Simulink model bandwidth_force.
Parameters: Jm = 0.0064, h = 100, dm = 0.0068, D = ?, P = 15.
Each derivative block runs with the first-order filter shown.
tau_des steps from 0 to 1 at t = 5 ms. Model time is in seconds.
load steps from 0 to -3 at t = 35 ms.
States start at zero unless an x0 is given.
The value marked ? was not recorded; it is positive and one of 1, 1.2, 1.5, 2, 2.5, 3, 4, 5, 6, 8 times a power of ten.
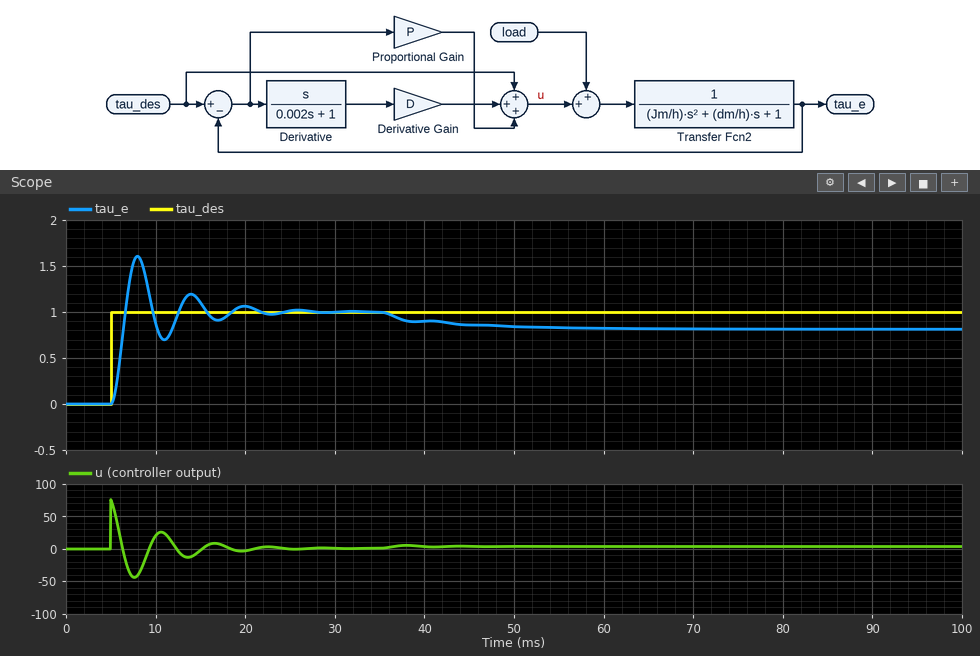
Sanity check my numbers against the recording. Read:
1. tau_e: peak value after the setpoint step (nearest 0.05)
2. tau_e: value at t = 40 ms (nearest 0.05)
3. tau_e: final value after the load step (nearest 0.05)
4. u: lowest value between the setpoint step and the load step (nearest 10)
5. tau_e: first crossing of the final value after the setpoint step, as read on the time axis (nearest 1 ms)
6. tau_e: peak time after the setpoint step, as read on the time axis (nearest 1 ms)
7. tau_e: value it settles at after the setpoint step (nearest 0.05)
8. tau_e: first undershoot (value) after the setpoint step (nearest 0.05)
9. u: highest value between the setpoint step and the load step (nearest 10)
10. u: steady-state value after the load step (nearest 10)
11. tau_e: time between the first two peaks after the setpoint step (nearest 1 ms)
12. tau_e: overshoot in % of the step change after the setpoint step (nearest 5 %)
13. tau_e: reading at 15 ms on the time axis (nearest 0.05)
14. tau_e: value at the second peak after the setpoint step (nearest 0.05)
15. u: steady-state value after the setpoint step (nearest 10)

1.60
0.90
0.80
-40
7 ms
8 ms
1.00
0.70
80
0
6 ms
60 %
1.10
1.20
0
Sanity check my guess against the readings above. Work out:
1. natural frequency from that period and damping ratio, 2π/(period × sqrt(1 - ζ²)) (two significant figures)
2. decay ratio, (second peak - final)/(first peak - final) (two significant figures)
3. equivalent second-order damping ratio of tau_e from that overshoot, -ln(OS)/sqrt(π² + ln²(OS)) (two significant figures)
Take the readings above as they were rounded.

1.1 rad/ms
0.33
0.16
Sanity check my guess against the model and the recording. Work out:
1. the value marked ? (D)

0.12
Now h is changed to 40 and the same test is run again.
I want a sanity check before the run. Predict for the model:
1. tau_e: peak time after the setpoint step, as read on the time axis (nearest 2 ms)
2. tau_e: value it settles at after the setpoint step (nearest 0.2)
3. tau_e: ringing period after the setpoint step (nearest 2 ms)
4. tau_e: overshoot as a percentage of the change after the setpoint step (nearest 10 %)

10 ms
1.0
10 ms
50 %
